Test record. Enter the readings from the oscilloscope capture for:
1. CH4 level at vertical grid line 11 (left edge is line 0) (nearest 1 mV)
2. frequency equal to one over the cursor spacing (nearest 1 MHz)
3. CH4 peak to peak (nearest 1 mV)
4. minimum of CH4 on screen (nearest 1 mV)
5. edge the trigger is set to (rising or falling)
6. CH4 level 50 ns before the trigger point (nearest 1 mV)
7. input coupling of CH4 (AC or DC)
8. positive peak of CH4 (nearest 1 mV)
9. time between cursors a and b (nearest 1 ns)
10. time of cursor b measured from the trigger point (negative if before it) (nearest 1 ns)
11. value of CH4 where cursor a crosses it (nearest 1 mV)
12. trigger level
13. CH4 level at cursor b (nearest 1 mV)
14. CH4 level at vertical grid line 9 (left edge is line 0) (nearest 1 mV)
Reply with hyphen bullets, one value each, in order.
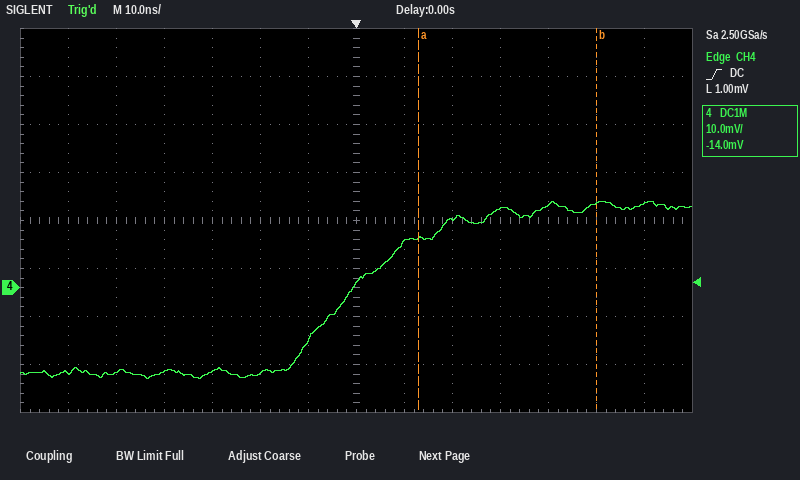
- 17 mV
- 27 MHz
- 37 mV
- -19 mV
- rising
- -18 mV
- DC
- 18 mV
- 37 ns
- +50 ns
- 10 mV
- 1.00 mV
- 18 mV
- 14 mV
